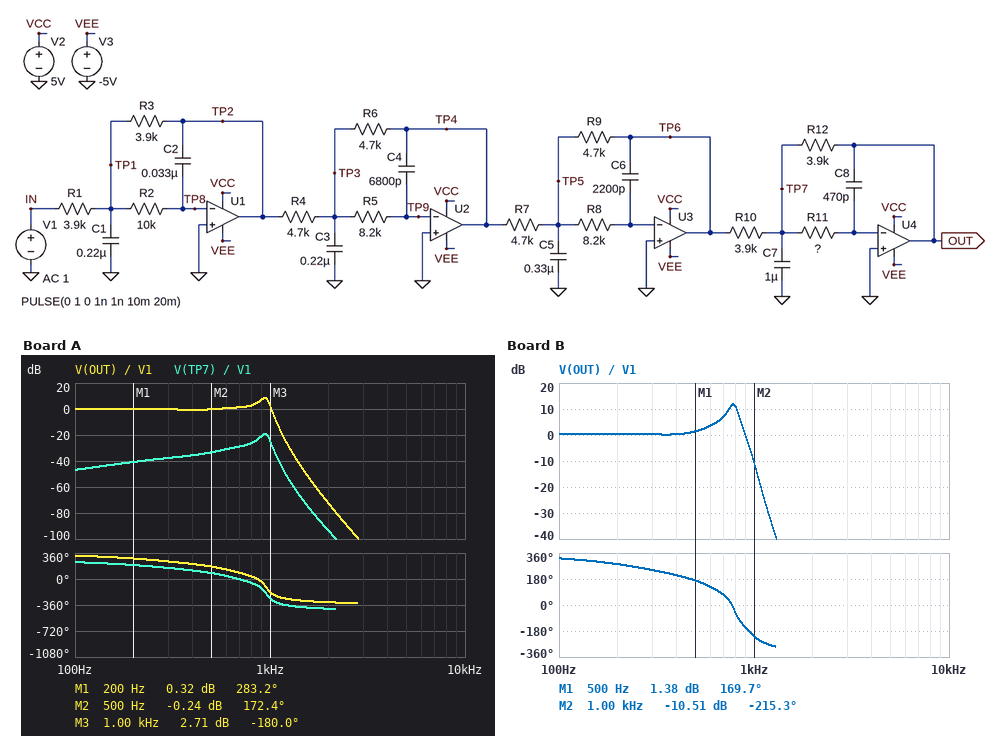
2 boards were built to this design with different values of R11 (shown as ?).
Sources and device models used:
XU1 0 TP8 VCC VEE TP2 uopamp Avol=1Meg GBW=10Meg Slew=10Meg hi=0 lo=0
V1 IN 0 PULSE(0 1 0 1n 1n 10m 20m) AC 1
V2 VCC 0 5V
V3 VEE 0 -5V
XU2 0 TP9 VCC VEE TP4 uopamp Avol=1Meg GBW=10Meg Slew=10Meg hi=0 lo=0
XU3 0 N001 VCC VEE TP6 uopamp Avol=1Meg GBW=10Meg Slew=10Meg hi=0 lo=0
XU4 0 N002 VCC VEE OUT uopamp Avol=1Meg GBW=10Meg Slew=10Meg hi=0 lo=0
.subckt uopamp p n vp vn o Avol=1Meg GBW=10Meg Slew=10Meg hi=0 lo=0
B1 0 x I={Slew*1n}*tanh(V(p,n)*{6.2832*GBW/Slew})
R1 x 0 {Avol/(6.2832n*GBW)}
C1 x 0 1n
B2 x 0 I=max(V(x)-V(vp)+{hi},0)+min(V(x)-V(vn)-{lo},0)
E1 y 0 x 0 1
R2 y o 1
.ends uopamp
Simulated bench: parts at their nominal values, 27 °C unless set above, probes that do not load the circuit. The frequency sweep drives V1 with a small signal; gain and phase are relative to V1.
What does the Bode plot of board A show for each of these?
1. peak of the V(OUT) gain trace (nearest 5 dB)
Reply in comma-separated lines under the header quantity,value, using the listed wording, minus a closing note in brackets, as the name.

quantity,value
peak of the V(OUT) gain trace,10 dB
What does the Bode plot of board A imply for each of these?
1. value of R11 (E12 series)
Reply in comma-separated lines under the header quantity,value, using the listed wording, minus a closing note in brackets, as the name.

quantity,value
value of R11,15 kΩ
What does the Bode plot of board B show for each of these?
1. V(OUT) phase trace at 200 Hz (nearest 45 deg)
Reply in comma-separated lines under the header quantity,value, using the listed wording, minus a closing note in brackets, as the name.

quantity,value
V(OUT) phase trace at 200 Hz,270 deg
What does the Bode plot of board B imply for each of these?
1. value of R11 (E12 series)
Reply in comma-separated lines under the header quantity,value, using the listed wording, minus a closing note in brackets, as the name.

quantity,value
value of R11,22 kΩ
